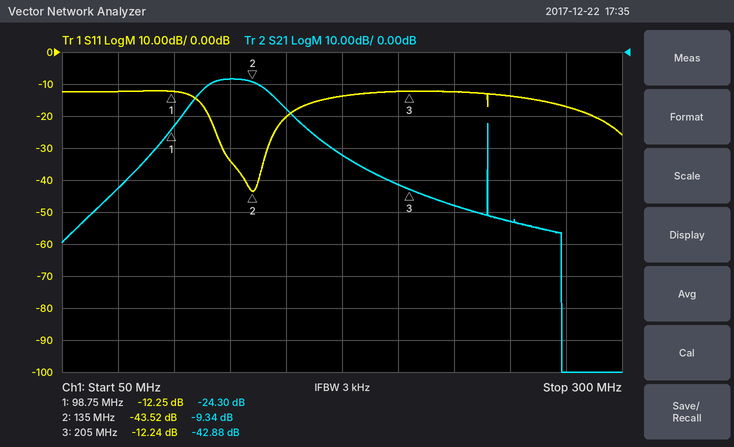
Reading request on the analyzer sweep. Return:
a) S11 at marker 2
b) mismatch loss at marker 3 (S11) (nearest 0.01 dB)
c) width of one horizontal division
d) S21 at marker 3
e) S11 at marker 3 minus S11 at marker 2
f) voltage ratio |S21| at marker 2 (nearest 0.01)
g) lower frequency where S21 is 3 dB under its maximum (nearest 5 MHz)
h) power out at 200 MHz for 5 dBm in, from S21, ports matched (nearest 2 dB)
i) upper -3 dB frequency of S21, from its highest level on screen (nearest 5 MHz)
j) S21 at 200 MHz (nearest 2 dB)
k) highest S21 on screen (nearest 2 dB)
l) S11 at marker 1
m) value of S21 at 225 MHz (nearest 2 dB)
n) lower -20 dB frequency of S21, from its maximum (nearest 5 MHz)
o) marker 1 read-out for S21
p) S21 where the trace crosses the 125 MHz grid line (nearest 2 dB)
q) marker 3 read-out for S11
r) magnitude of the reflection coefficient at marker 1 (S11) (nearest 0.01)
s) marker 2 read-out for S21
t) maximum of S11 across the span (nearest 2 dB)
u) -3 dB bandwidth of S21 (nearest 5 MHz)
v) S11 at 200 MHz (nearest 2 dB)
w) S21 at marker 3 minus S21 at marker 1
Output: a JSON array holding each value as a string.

["-43.52 dB", "0.27 dB", "25 MHz", "-42.88 dB", "31.28 dB", "0.34", "115 MHz", "-36 dBm", "140 MHz", "-42 dB", "-8 dB", "-12.25 dB", "-48 dB", "95 MHz", "-24.30 dB", "-8 dB", "-12.24 dB", "0.24", "-9.34 dB", "-12 dB", "25 MHz", "-12 dB", "-18.58 dB"]
